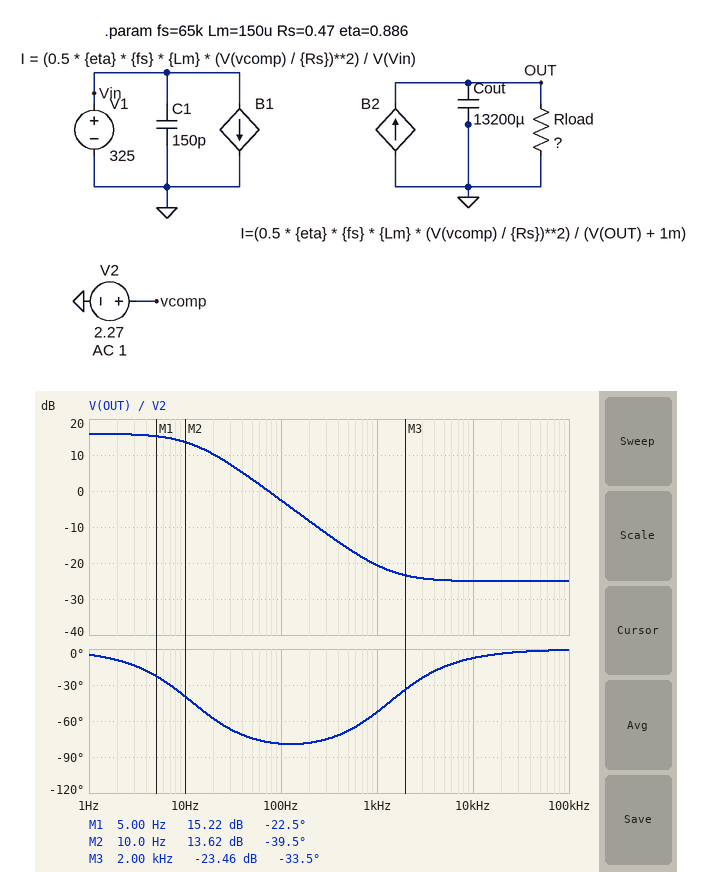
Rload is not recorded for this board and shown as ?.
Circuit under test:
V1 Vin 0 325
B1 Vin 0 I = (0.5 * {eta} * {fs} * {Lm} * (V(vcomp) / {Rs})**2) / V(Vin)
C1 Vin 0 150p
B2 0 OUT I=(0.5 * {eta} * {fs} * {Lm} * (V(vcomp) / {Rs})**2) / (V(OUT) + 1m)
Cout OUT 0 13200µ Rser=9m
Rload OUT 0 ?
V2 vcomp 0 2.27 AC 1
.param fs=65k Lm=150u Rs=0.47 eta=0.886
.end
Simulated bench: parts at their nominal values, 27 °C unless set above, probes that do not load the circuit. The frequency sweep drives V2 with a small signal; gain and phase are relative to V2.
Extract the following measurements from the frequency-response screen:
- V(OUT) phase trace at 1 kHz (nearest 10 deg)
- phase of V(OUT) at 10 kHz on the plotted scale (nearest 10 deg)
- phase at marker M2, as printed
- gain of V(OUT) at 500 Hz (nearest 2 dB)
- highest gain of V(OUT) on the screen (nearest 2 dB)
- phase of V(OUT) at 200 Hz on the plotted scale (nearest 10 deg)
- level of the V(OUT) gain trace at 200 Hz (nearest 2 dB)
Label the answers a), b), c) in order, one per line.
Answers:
a) -50 deg
b) -10 deg
c) -39.5 deg
d) -16 dB
e) 16 dB
f) -80 deg
g) -8 dB
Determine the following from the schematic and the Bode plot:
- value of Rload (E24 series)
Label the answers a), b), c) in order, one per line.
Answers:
a) 2 Ω
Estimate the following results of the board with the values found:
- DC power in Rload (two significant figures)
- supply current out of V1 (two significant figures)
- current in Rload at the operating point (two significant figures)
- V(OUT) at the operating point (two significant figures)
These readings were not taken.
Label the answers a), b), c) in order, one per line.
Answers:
a) 100 W
b) 310 mA
c) 7.1 A
d) 14 V
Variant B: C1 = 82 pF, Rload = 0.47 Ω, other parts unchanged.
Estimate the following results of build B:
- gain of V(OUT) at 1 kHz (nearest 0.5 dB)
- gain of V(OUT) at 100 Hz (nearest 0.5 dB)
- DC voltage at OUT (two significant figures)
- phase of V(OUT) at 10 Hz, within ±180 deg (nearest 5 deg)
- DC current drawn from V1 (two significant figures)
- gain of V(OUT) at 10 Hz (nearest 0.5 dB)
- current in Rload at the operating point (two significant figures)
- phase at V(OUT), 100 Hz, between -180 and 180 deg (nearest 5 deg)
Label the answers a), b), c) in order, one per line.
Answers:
a) -14.5 dB
b) 2.5 dB
c) 6.9 V
d) -10 deg
e) 310 mA
f) 9.5 dB
g) 15 A
h) -60 deg
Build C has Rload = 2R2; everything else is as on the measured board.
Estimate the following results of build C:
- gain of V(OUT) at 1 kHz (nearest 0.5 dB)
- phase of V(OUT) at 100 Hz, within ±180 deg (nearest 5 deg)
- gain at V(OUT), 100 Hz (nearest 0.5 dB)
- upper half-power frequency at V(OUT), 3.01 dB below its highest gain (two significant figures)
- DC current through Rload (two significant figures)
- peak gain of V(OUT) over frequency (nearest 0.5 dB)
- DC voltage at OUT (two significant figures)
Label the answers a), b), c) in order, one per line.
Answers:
a) -21.0 dB
b) -80 deg
c) -3.0 dB
d) 11 Hz
e) 6.8 A
f) 16.5 dB
g) 15 V
